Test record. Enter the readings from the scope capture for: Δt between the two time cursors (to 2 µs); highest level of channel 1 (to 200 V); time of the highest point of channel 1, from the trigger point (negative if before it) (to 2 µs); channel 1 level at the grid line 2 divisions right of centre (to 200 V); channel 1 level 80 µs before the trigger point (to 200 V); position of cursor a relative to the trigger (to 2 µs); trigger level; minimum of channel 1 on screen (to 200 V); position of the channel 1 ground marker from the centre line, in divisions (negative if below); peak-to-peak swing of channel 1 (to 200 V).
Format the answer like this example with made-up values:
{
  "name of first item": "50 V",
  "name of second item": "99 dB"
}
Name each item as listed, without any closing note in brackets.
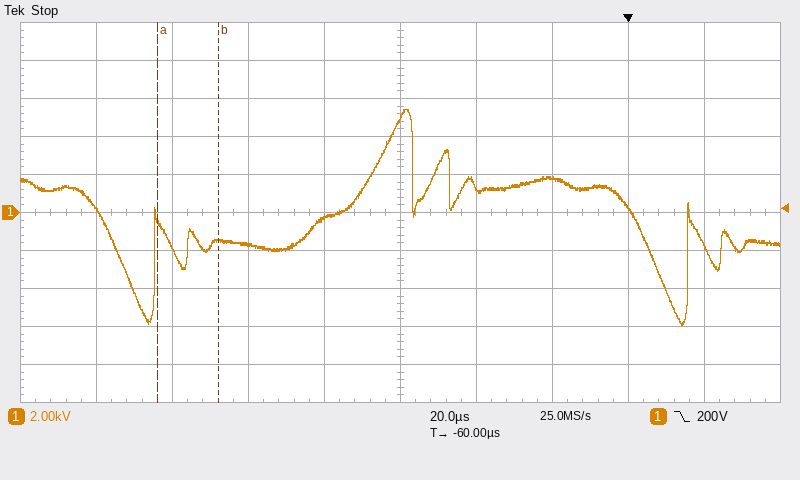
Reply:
{
  "Δt between the two time cursors": "16 µs",
  "highest level of channel 1": "5.4 kV",
  "time of the highest point of channel 1, from the trigger point (negative if before it)": "-58 µs",
  "channel 1 level at the grid line 2 divisions right of centre": "1.8 kV",
  "channel 1 level 80 µs before the trigger point": "-400 V",
  "position of cursor a relative to the trigger": "-124 µs",
  "trigger level": "200 V",
  "minimum of channel 1 on screen": "-6.0 kV",
  "position of the channel 1 ground marker from the centre line, in divisions": "0.0 div",
  "peak-to-peak swing of channel 1": "11.4 kV"
}
